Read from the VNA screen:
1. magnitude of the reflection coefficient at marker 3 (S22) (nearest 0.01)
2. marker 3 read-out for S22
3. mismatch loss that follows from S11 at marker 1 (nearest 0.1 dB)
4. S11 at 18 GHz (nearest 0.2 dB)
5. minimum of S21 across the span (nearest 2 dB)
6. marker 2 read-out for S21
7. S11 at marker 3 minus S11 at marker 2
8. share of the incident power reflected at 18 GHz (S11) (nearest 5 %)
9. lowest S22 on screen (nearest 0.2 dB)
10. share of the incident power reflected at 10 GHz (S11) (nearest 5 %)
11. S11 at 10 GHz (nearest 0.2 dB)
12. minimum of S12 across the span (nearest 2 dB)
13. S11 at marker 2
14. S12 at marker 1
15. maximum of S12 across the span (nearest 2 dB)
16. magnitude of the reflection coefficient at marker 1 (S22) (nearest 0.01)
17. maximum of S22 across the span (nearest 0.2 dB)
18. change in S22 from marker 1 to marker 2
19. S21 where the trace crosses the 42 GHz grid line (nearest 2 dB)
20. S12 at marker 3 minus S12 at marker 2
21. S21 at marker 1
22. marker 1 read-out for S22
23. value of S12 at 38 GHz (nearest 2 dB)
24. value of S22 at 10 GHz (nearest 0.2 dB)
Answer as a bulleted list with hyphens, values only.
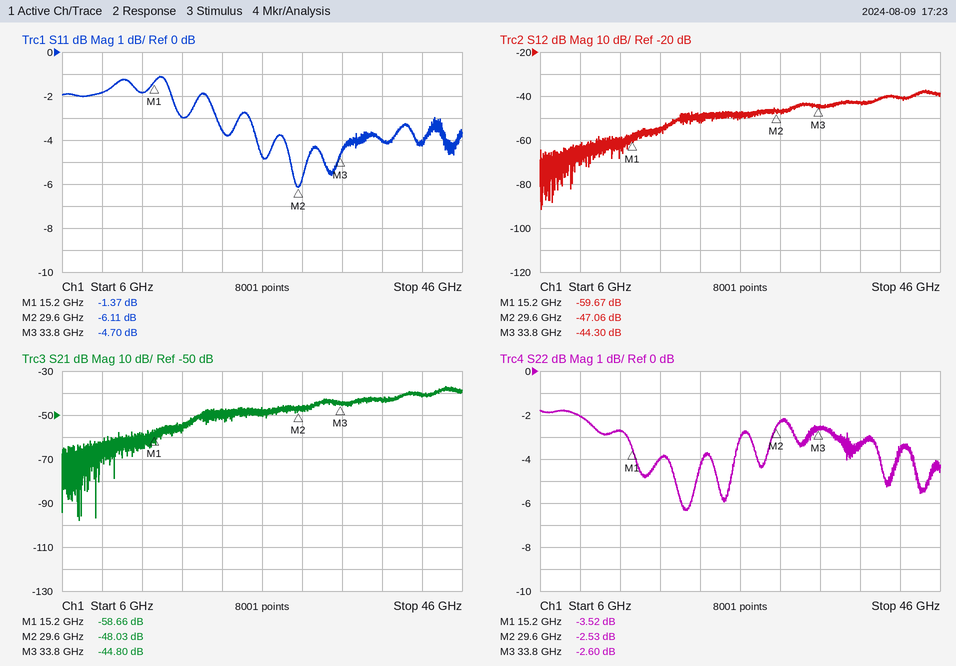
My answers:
- 0.74
- -2.60 dB
- 5.7 dB
- -3.0 dB
- -98 dB
- -48.03 dB
- 1.41 dB
- 50 %
- -6.4 dB
- 65 %
- -1.8 dB
- -92 dB
- -6.11 dB
- -59.67 dB
- -38 dB
- 0.67
- -1.8 dB
- 0.99 dB
- -40 dB
- 2.76 dB
- -58.66 dB
- -3.52 dB
- -42 dB
- -2.0 dB
